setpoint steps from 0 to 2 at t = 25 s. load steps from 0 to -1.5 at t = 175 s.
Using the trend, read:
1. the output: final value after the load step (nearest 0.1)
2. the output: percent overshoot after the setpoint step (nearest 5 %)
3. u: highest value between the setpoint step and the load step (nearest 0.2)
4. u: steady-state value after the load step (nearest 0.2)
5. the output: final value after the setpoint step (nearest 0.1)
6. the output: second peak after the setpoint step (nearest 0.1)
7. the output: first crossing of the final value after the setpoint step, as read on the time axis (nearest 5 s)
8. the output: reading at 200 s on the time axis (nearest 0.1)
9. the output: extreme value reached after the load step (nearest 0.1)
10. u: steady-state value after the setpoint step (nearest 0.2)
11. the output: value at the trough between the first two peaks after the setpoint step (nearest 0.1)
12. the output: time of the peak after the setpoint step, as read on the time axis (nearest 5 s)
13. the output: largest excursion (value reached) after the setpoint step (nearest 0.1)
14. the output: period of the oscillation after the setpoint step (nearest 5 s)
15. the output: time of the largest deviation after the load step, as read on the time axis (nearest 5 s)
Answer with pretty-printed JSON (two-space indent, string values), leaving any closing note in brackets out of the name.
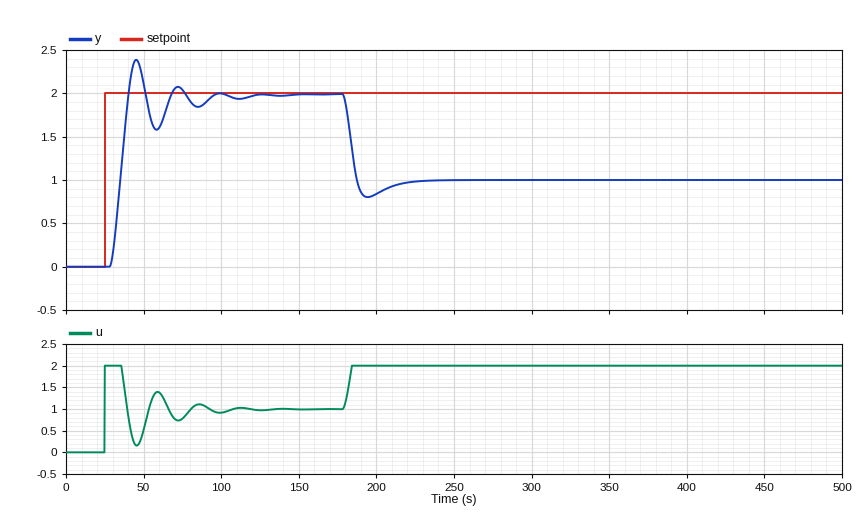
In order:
{
  "the output: final value after the load step": "1.0",
  "the output: percent overshoot after the setpoint step": "20 %",
  "u: highest value between the setpoint step and the load step": "2.0",
  "u: steady-state value after the load step": "2.0",
  "the output: final value after the setpoint step": "2.0",
  "the output: second peak after the setpoint step": "2.1",
  "the output: first crossing of the final value after the setpoint step, as read on the time axis": "40 s",
  "the output: reading at 200 s on the time axis": "0.8",
  "the output: extreme value reached after the load step": "0.8",
  "u: steady-state value after the setpoint step": "1.0",
  "the output: value at the trough between the first two peaks after the setpoint step": "1.6",
  "the output: time of the peak after the setpoint step, as read on the time axis": "45 s",
  "the output: largest excursion (value reached) after the setpoint step": "2.4",
  "the output: period of the oscillation after the setpoint step": "25 s",
  "the output: time of the largest deviation after the load step, as read on the time axis": "195 s"
}
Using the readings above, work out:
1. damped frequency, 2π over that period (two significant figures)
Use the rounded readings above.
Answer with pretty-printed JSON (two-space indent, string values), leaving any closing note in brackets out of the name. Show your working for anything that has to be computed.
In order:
{
  "damped frequency, 2π over that period": "2π / 25 = 0.25 rad/s"
}
